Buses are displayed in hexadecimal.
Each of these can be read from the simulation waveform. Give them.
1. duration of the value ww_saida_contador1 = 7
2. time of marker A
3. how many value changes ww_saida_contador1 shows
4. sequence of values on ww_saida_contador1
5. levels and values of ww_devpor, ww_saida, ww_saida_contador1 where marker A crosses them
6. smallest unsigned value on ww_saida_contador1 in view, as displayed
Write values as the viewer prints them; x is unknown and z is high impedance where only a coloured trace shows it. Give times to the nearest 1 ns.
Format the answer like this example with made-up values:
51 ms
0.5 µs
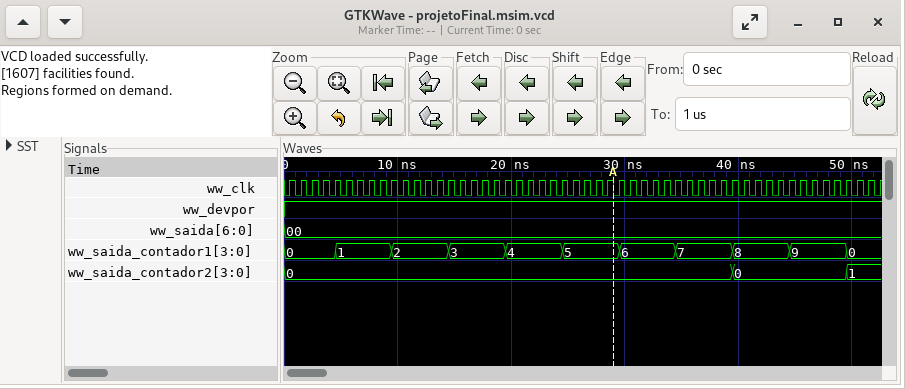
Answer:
5 ns
29 ns
10
0, 1, 2, 3, 4, 5, 6, 7, 8, 9, 0
ww_devpor=1, ww_saida=00, ww_saida_contador1=5
0
